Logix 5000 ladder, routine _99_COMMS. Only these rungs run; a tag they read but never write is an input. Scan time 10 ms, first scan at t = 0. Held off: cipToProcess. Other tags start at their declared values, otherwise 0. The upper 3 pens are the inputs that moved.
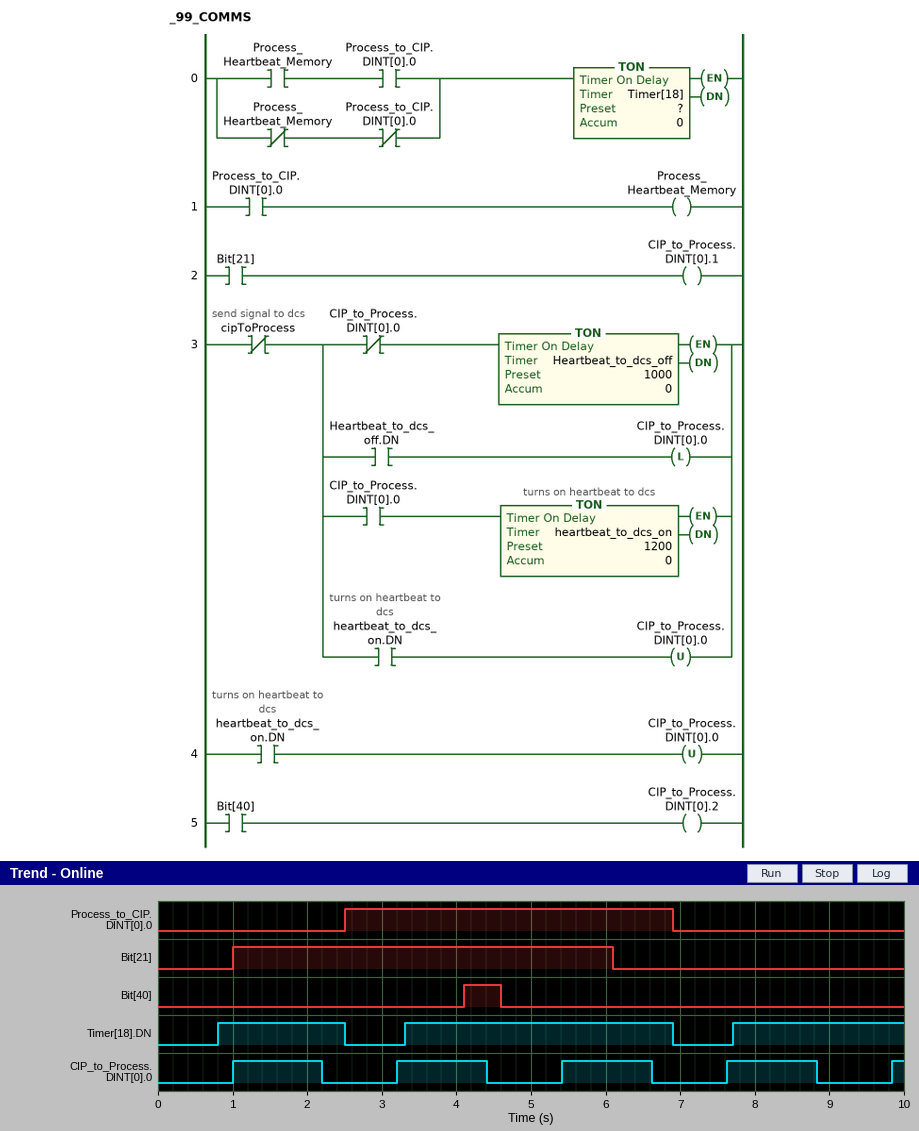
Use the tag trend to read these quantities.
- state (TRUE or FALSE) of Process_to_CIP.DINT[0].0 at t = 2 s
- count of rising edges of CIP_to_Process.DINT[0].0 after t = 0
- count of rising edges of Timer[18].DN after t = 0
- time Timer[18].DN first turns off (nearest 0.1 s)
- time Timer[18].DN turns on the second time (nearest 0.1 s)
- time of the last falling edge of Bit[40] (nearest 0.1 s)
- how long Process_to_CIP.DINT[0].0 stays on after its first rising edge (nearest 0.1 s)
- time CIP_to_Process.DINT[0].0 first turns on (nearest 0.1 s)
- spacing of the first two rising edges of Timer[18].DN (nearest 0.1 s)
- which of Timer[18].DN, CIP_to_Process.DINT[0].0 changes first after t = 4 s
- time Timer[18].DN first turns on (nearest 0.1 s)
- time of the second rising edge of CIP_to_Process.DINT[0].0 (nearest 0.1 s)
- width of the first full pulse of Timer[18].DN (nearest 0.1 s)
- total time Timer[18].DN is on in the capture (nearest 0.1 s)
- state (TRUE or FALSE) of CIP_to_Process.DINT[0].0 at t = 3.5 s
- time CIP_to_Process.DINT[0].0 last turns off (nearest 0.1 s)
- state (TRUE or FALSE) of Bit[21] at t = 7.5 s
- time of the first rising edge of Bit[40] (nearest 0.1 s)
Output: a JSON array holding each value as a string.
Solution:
["FALSE", "5", "3", "2.5 s", "3.3 s", "4.6 s", "4.4 s", "1.0 s", "2.5 s", "CIP_to_Process.DINT[0].0", "0.8 s", "3.2 s", "1.7 s", "7.6 s", "TRUE", "8.8 s", "FALSE", "4.1 s"]
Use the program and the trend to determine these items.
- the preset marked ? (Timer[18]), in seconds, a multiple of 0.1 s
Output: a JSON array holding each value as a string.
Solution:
["0.8 s"]
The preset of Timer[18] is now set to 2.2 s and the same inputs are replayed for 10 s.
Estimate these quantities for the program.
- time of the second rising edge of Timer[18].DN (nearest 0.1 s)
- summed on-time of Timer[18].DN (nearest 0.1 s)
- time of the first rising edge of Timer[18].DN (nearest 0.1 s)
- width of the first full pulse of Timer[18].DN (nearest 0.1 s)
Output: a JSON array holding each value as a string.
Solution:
["4.7 s", "3.4 s", "2.2 s", "0.3 s"]
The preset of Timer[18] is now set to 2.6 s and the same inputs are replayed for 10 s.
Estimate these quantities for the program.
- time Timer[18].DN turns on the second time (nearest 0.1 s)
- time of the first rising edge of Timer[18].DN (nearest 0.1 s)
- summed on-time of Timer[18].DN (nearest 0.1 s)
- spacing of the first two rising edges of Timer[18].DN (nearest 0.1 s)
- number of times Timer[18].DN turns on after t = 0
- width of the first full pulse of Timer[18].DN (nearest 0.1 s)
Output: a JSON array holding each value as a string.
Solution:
["9.5 s", "5.1 s", "2.3 s", "4.4 s", "2", "1.8 s"]
